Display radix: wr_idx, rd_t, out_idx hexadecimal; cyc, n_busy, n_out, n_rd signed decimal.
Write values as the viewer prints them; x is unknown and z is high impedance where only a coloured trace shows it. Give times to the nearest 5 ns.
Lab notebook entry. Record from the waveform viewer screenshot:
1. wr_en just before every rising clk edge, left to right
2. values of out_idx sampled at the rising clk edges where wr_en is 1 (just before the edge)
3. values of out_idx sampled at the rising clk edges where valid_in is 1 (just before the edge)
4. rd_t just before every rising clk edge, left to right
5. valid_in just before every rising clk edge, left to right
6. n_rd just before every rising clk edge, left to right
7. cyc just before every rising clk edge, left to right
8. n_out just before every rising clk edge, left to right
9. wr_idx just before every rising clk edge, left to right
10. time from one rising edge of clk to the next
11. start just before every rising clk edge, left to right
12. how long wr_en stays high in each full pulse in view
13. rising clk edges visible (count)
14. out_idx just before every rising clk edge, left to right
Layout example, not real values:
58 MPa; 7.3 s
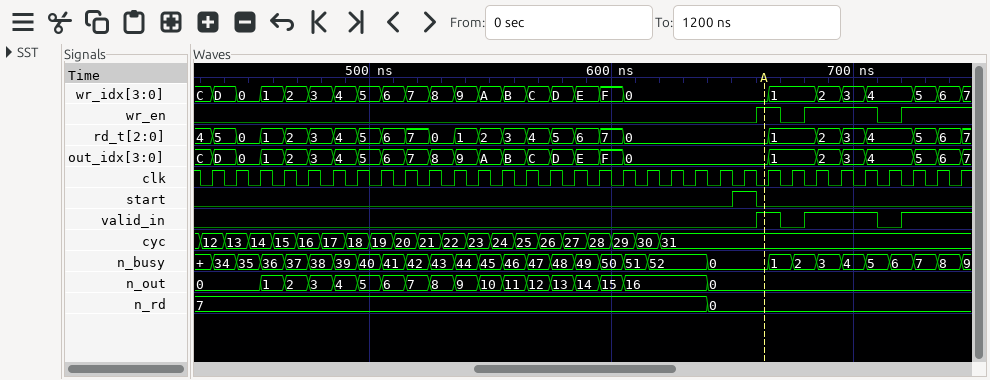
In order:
0 0 0 0 0 0 0 0 0 0 0 0 0 0 0 0 0 0 0 0 0 0 0 1 0 1 1 1 0 1 1 1; 0, 1, 2, 3, 4, 5, 6; 0, 1, 2, 3, 4, 5, 6; 4, 5, 0, 1, 2, 3, 4, 5, 6, 7, 0, 1, 2, 3, 4, 5, 6, 7, 0, 0, 0, 0, 0, 0, 1, 1, 2, 3, 4, 4, 5, 6; 0 0 0 0 0 0 0 0 0 0 0 0 0 0 0 0 0 0 0 0 0 0 0 1 0 1 1 1 0 1 1 1; 7, 7, 7, 7, 7, 7, 7, 7, 7, 7, 7, 7, 7, 7, 7, 7, 7, 7, 7, 7, 7, 0, 0, 0, 0, 0, 0, 0, 0, 0, 0, 0; 12, 13, 14, 15, 16, 17, 18, 19, 20, 21, 22, 23, 24, 25, 26, 27, 28, 29, 30, 31, 31, 31, 31, 31, 31, 31, 31, 31, 31, 31, 31, 31; 0, 0, 0, 1, 2, 3, 4, 5, 6, 7, 8, 9, 10, 11, 12, 13, 14, 15, 16, 16, 16, 0, 0, 0, 0, 0, 0, 0, 0, 0, 0, 0; C, D, 0, 1, 2, 3, 4, 5, 6, 7, 8, 9, A, B, C, D, E, F, 0, 0, 0, 0, 0, 0, 1, 1, 2, 3, 4, 4, 5, 6; 10 ns; 0 0 0 0 0 0 0 0 0 0 0 0 0 0 0 0 0 0 0 0 0 0 1 0 0 0 0 0 0 0 0 0; 10 ns, 30 ns; 32; C, D, 0, 1, 2, 3, 4, 5, 6, 7, 8, 9, A, B, C, D, E, F, 0, 0, 0, 0, 0, 0, 1, 1, 2, 3, 4, 4, 5, 6
